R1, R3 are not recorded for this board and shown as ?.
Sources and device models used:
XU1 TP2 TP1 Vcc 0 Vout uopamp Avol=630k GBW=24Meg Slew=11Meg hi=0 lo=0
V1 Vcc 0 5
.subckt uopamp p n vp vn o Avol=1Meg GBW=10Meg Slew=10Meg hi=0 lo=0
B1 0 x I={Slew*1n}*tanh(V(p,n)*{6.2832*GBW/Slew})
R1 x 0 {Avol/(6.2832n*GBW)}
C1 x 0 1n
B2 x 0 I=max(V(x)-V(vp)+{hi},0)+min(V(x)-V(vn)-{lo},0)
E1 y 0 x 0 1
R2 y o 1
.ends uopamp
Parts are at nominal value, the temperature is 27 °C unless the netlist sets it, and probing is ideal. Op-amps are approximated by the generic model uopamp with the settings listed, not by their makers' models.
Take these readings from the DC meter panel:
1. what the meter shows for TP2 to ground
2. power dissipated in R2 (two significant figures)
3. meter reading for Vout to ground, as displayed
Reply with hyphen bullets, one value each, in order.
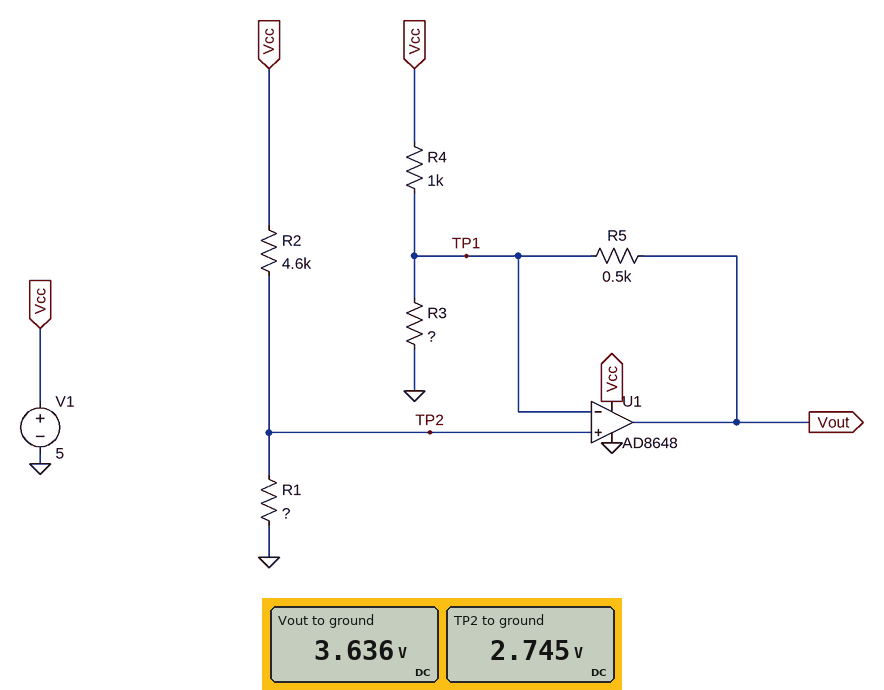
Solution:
- 2.745 V
- 1.1 mW
- 3.636 V
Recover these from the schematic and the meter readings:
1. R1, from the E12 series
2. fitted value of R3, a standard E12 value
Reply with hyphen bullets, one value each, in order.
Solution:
- 5.6 kΩ
- 680 Ω
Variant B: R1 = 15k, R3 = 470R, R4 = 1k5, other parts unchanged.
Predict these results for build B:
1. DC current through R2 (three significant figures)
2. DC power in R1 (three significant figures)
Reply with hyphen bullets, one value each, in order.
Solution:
- 255 µA
- 976 µW
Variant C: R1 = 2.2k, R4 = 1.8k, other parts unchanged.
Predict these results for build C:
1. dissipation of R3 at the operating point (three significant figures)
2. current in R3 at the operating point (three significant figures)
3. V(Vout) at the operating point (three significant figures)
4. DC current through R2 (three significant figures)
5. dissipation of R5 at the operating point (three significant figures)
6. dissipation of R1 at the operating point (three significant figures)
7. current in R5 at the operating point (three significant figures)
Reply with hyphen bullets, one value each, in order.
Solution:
- 3.85 mW
- 2.38 mA
- 1.87 V
- 735 µA
- 125 µW
- 1.19 mW
- 500 µA
